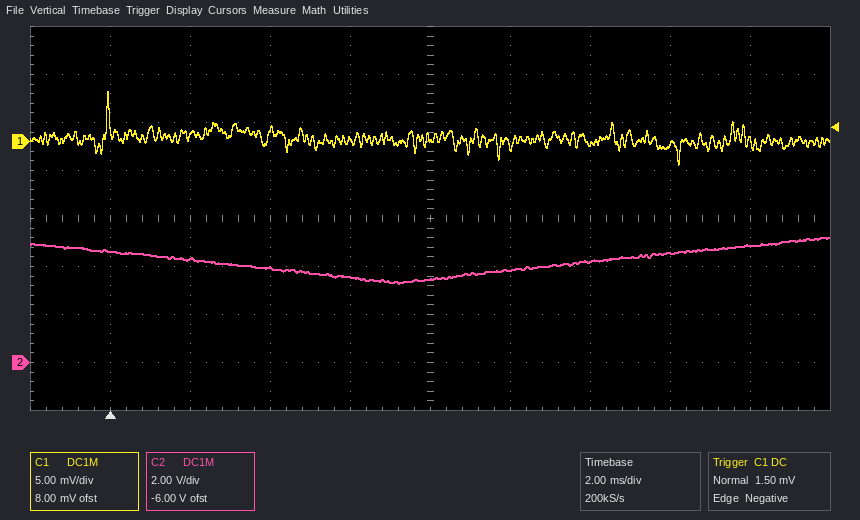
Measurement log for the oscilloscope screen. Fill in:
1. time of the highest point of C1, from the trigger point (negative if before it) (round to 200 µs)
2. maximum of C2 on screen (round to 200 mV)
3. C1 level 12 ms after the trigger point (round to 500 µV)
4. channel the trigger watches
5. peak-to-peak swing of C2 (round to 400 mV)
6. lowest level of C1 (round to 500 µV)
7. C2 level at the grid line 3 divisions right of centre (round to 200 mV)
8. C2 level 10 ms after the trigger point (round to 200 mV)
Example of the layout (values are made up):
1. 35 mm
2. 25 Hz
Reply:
1. 0.0 ms
2. 5.2 V
3. 0.0 mV
4. C1
5. 2.0 V
6. -2.5 mV
7. 4.6 V
8. 3.8 V
